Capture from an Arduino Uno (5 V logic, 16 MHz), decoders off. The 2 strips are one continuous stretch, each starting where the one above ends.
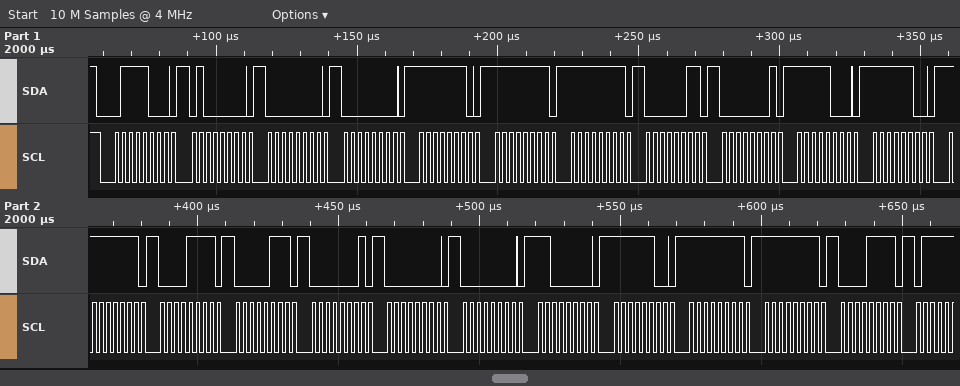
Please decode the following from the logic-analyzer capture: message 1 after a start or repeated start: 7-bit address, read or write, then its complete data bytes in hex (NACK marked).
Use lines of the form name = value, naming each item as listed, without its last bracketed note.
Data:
message 1 after a start or repeated start: 7-bit address, read or write, then its complete data bytes in hex = 0x3C write: 40 00 00 FE FF FF 03 01 F8 FC FF 0F 07 01 00 00 C0 FC FF FF 0F
